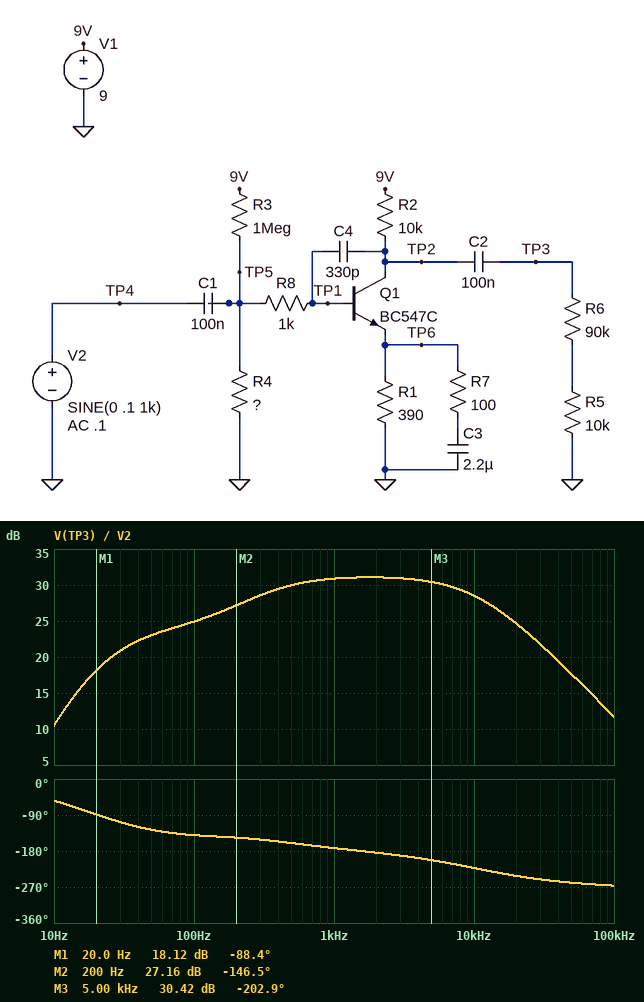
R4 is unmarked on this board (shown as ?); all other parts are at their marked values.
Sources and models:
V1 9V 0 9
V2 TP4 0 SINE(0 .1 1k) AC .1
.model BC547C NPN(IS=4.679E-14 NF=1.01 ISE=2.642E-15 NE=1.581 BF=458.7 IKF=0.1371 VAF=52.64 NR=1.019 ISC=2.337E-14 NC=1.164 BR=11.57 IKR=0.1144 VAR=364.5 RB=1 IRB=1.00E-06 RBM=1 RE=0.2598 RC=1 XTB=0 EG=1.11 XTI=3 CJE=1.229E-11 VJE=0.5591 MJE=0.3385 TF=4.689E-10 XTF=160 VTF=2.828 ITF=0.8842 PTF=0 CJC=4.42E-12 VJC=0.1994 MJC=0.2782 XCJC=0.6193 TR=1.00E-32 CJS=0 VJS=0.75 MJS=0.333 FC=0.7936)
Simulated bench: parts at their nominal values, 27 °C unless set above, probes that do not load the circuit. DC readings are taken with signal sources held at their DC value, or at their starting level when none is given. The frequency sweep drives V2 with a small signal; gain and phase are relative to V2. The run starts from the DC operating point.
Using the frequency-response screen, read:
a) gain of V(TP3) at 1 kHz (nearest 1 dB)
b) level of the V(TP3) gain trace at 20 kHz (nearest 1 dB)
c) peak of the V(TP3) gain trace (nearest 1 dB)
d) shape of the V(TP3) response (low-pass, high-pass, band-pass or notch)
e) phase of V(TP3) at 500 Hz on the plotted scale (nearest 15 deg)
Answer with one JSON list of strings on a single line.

["31 dB", "25 dB", "31 dB", "band-pass", "-165 deg"]
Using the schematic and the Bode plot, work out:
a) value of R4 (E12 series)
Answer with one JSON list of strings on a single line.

["82 kΩ"]
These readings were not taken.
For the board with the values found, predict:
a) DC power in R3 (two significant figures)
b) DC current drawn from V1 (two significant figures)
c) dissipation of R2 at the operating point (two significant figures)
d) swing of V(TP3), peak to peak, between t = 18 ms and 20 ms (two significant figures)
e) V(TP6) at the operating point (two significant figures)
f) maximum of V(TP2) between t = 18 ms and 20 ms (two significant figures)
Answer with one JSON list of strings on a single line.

["70 µW", "200 µA", "380 µW", "5.6 V", "77 mV", "8.7 V"]
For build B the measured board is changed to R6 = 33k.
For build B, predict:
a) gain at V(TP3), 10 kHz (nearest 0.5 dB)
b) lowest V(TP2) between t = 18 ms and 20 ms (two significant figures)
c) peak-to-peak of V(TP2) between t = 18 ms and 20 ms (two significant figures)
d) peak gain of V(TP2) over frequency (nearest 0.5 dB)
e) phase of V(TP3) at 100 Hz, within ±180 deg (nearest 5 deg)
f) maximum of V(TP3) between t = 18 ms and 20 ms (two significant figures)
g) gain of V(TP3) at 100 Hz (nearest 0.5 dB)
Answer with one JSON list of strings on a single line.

["28.0 dB", "3.4 V", "5.1 V", "30.0 dB", "-130 deg", "1.8 V", "23.5 dB"]
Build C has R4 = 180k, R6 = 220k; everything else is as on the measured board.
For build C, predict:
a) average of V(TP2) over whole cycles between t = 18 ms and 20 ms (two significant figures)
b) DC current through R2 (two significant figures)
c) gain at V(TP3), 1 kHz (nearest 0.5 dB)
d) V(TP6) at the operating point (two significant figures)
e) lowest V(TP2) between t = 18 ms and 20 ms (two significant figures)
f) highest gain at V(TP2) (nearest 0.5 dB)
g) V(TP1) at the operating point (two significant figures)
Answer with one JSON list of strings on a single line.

["4.1 V", "850 µA", "22.0 dB", "330 mV", "270 mV", "25.0 dB", "950 mV"]
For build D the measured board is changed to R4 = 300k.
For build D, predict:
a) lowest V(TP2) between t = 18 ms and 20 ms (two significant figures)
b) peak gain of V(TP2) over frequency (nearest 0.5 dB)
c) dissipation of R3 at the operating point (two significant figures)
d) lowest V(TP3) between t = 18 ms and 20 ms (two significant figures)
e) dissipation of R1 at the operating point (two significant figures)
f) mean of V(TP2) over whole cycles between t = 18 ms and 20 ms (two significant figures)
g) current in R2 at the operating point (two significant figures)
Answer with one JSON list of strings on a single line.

["280 mV", "15.5 dB", "65 µW", "-2.9 V", "290 µW", "3.7 V", "860 µA"]
